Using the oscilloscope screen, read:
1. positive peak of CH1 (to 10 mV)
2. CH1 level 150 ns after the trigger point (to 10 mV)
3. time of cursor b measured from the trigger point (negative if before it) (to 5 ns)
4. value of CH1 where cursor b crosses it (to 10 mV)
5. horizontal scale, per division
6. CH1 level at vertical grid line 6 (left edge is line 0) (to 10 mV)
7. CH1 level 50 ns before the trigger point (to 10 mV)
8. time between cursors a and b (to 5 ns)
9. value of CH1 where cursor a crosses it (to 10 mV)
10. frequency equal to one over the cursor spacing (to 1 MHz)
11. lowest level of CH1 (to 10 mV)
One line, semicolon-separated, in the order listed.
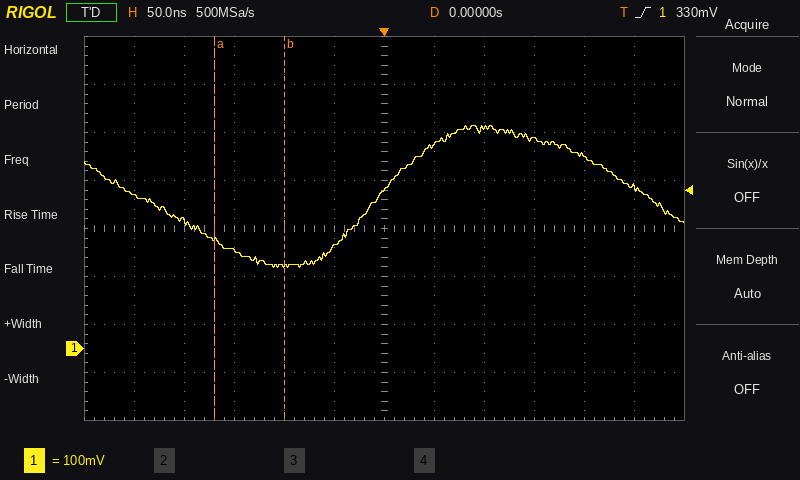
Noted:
460 mV; 440 mV; -100 ns; 170 mV; 50 ns; 330 mV; 210 mV; 70 ns; 230 mV; 14 MHz; 170 mV
